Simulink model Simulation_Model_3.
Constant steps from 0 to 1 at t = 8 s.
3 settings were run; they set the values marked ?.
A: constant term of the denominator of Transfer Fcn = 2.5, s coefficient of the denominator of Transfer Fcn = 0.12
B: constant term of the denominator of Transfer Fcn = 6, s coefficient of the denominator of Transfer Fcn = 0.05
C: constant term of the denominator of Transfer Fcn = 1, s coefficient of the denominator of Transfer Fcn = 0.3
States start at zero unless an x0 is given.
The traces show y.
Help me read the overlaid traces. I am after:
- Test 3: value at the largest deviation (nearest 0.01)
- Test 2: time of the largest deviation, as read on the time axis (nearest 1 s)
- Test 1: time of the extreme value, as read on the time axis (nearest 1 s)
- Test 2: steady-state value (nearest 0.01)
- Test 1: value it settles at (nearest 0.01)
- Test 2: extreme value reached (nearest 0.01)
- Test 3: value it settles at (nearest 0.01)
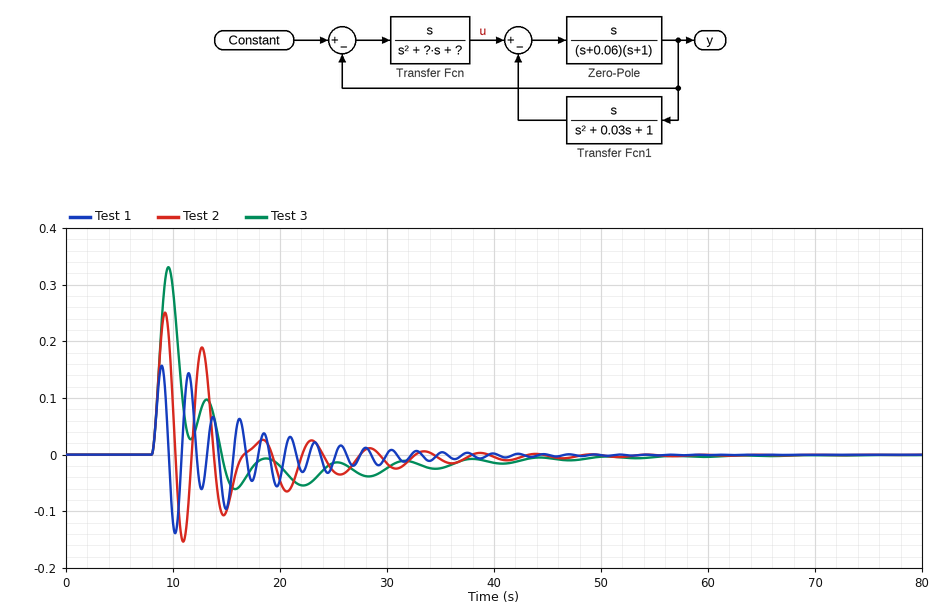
0.33
9 s
9 s
0.00
0.00
0.25
0.00
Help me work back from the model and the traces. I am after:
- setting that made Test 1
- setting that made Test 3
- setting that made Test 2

B
C
A
